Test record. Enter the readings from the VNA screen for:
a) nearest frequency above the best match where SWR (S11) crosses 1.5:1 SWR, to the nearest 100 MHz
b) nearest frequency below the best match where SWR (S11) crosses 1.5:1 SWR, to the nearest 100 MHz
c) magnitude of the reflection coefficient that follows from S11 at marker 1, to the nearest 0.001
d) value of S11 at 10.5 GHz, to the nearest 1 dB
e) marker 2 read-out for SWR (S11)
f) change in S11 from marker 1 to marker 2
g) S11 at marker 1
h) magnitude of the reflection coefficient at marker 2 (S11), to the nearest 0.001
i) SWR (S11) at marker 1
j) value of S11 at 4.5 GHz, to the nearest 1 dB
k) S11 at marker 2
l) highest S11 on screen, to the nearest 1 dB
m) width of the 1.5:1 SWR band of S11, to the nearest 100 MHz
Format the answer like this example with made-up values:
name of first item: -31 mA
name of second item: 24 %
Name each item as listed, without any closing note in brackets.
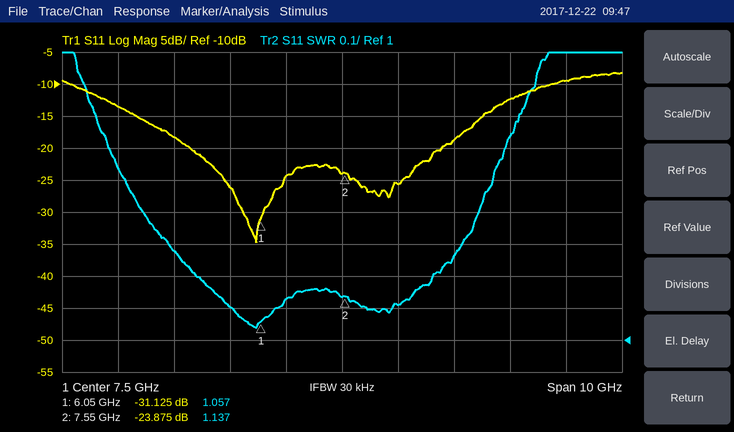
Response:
nearest frequency above the best match where SWR (S11) crosses 1.5:1 SWR, to the nearest 100 MHz: 10.2 GHz
nearest frequency below the best match where SWR (S11) crosses 1.5:1 SWR, to the nearest 100 MHz: 3.6 GHz
magnitude of the reflection coefficient that follows from S11 at marker 1, to the nearest 0.001: 0.028
value of S11 at 10.5 GHz, to the nearest 1 dB: -12 dB
marker 2 read-out for SWR: 1.137
change in S11 from marker 1 to marker 2: 7.250 dB
S11 at marker 1: -31.125 dB
magnitude of the reflection coefficient at marker 2 (S11), to the nearest 0.001: 0.064
SWR (S11) at marker 1: 1.057
value of S11 at 4.5 GHz, to the nearest 1 dB: -18 dB
S11 at marker 2: -23.875 dB
highest S11 on screen, to the nearest 1 dB: -8 dB
width of the 1.5:1 SWR band of S11, to the nearest 100 MHz: 6.6 GHz
